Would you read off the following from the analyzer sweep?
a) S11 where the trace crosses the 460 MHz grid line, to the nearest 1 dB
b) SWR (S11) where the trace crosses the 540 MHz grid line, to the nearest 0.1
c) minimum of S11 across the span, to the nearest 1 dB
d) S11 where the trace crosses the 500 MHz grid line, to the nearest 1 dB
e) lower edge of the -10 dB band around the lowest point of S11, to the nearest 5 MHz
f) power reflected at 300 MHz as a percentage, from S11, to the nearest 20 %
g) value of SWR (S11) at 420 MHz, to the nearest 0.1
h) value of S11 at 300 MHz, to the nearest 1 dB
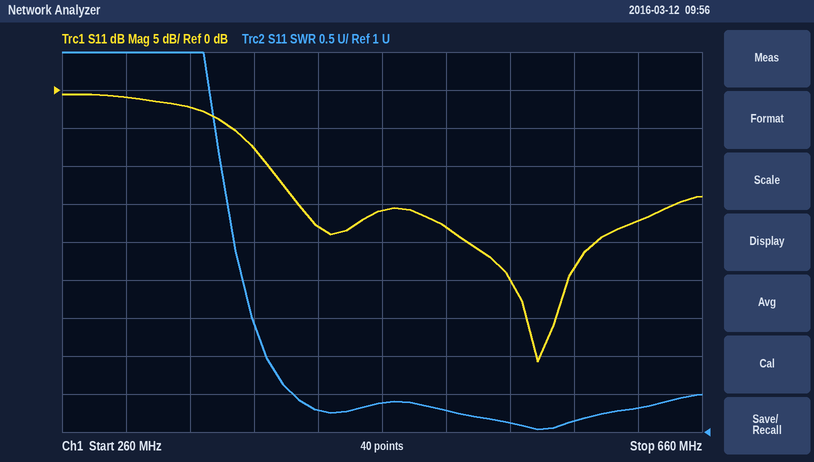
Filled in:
-16 dB
1.1
-36 dB
-18 dB
390 MHz
80 %
1.3
-1 dB
